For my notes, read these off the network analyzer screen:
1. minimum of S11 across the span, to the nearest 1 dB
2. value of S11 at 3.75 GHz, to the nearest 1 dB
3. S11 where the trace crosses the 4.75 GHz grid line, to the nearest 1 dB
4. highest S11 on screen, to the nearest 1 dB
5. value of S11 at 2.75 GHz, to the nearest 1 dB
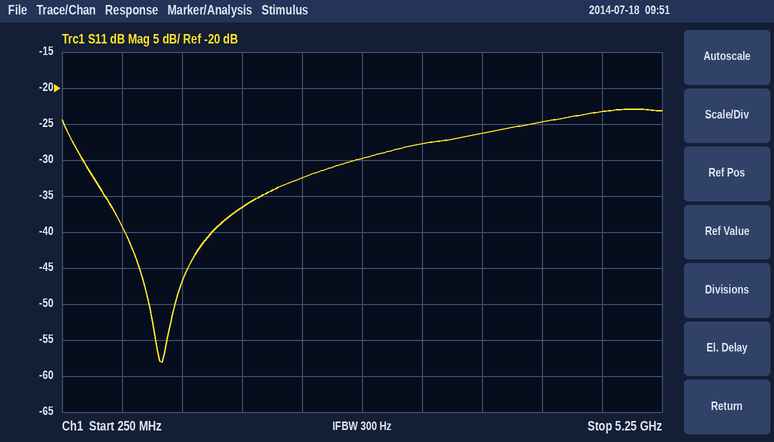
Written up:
-58 dB
-26 dB
-23 dB
-23 dB
-30 dB
